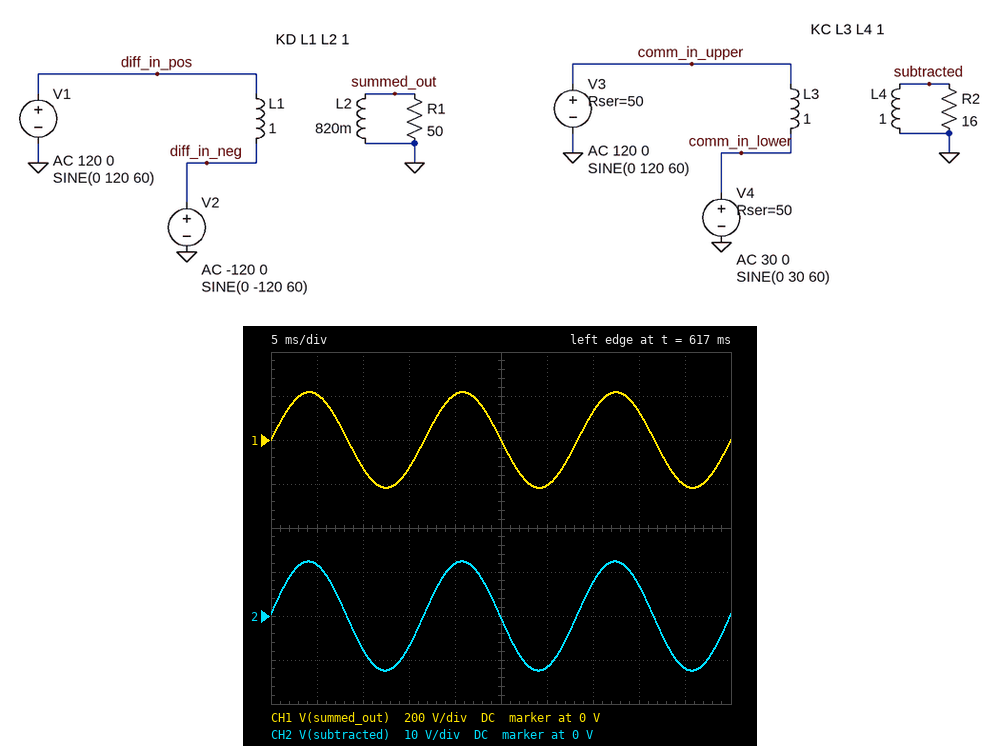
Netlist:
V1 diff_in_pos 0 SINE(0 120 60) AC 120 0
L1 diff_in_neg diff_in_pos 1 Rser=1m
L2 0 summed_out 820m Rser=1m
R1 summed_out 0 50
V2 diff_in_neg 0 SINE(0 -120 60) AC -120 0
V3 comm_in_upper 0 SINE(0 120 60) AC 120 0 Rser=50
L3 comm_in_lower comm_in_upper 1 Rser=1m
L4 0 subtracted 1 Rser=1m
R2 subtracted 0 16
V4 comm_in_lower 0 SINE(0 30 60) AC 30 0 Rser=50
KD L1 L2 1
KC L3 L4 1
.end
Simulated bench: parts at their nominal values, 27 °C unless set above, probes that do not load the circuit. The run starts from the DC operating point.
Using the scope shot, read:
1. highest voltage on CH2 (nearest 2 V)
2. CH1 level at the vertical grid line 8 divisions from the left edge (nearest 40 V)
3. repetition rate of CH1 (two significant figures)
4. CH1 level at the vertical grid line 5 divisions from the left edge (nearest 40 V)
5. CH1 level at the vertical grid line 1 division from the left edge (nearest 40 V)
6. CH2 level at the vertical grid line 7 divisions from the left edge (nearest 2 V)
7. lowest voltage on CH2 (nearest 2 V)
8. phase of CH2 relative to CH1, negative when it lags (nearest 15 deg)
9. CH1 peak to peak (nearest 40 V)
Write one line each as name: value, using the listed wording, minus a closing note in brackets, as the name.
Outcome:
highest voltage on CH2: 12 V
CH1 level at the vertical grid line 8 divisions from the left edge: 120 V
repetition rate of CH1: 60 Hz
CH1 level at the vertical grid line 5 divisions from the left edge: 0 V
CH1 level at the vertical grid line 1 division from the left edge: 200 V
CH2 level at the vertical grid line 7 divisions from the left edge: 8 V
lowest voltage on CH2: -12 V
phase of CH2 relative to CH1, negative when it lags: 0 deg
CH1 peak to peak: 440 V
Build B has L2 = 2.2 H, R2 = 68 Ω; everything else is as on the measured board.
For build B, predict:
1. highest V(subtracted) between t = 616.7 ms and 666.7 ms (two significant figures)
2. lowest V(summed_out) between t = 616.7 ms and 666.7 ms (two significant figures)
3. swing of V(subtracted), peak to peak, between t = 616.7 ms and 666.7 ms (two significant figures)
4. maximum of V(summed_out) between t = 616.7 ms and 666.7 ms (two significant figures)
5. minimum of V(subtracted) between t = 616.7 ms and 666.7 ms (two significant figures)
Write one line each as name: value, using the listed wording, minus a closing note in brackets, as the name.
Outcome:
highest V(subtracted) between t = 616.7 ms and 666.7 ms: 36 V
lowest V(summed_out) between t = 616.7 ms and 666.7 ms: -360 V
swing of V(subtracted), peak to peak, between t = 616.7 ms and 666.7 ms: 72 V
maximum of V(summed_out) between t = 616.7 ms and 666.7 ms: 360 V
minimum of V(subtracted) between t = 616.7 ms and 666.7 ms: -36 V
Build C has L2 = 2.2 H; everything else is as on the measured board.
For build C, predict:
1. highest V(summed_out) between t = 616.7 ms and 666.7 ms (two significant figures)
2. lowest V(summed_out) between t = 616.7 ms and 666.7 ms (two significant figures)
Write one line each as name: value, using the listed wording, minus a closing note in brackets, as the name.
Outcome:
highest V(summed_out) between t = 616.7 ms and 666.7 ms: 360 V
lowest V(summed_out) between t = 616.7 ms and 666.7 ms: -360 V
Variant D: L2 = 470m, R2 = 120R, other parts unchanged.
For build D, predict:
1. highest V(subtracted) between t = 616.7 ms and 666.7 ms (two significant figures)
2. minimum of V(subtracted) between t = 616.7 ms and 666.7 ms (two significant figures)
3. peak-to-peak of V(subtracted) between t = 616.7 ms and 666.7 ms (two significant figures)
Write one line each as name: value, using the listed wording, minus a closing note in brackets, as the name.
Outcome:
highest V(subtracted) between t = 616.7 ms and 666.7 ms: 49 V
minimum of V(subtracted) between t = 616.7 ms and 666.7 ms: -49 V
peak-to-peak of V(subtracted) between t = 616.7 ms and 666.7 ms: 97 V
